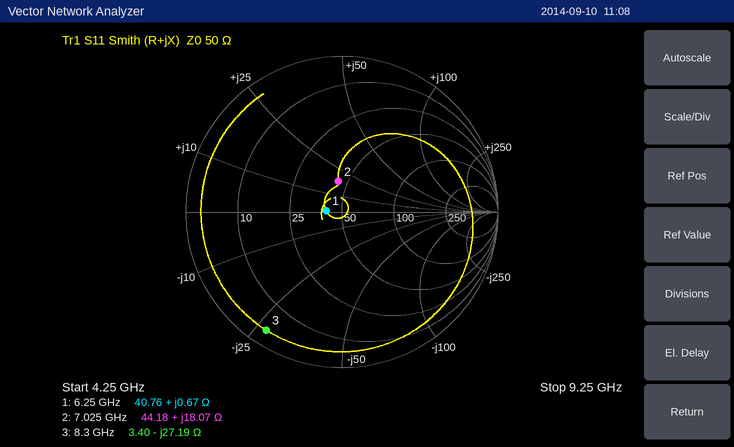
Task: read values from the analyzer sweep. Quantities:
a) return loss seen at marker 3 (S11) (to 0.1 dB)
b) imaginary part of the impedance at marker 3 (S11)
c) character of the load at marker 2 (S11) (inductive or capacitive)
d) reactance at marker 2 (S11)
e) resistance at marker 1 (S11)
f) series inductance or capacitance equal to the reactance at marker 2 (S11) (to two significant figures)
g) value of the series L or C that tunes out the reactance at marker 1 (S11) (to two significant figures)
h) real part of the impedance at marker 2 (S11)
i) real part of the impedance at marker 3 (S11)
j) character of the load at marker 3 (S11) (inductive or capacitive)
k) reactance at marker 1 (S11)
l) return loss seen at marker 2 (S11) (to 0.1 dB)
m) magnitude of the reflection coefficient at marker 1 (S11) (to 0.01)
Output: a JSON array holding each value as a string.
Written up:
["0.9 dB", "-27.19 Ω", "inductive", "+18.07 Ω", "40.76 Ω", "410 pH", "38 pF", "44.18 Ω", "3.40 Ω", "capacitive", "+0.67 Ω", "14.1 dB", "0.10"]
